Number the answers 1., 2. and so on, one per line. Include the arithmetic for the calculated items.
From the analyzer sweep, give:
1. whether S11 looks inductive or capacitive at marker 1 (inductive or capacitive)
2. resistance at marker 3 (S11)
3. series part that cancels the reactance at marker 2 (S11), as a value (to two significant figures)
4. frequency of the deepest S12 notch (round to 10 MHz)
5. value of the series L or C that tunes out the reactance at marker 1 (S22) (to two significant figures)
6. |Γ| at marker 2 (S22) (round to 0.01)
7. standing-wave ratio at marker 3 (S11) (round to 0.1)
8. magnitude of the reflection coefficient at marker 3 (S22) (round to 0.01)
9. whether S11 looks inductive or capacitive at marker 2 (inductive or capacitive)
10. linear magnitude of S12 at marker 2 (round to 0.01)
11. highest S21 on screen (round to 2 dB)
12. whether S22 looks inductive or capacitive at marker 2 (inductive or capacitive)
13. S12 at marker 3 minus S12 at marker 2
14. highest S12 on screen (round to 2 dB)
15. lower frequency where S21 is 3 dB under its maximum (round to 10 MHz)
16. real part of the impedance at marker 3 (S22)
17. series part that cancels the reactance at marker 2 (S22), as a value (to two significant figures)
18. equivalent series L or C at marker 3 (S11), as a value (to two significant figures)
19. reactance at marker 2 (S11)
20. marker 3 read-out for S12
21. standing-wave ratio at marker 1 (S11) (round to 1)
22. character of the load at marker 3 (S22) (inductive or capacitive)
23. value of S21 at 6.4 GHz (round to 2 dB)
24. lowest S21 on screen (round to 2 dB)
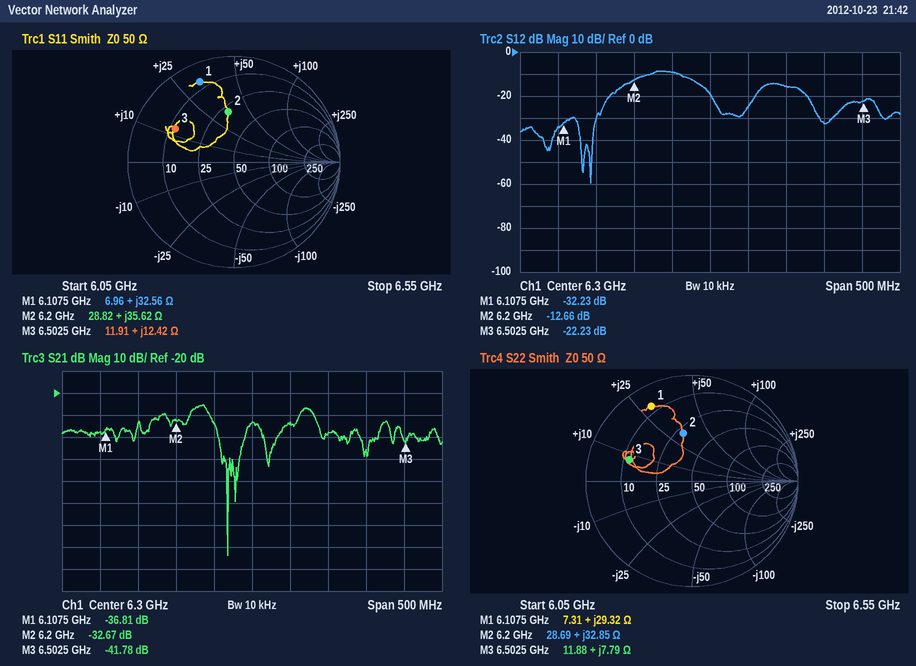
1. inductive
2. 11.91 Ω
3. C = 1/(2π × 6.2 GHz × 35.62 Ω) ≈ 721 fF, so 720 fF to two significant figures
4. 6.14 GHz
5. C = 1/(2π × 6.1075 GHz × 29.32 Ω) ≈ 889 fF, so 890 fF to two significant figures
6. 0.46
7. 4.5
8. 0.62
9. inductive
10. 10^(-12.66/20) ≈ 0.23
11. -26 dB
12. inductive
13. -22.23 − (-12.66) = -9.57 dB
14. -8 dB
15. 6.22 GHz
16. 11.88 Ω
17. C = 1/(2π × 6.2 GHz × 32.85 Ω) ≈ 781 fF, so 780 fF to two significant figures
18. L = 12.42 Ω/(2π × 6.5025 GHz) ≈ 304 pH, so 300 pH to two significant figures
19. +35.62 Ω
20. -22.23 dB
21. 10
22. inductive
23. -38 dB
24. -94 dB
